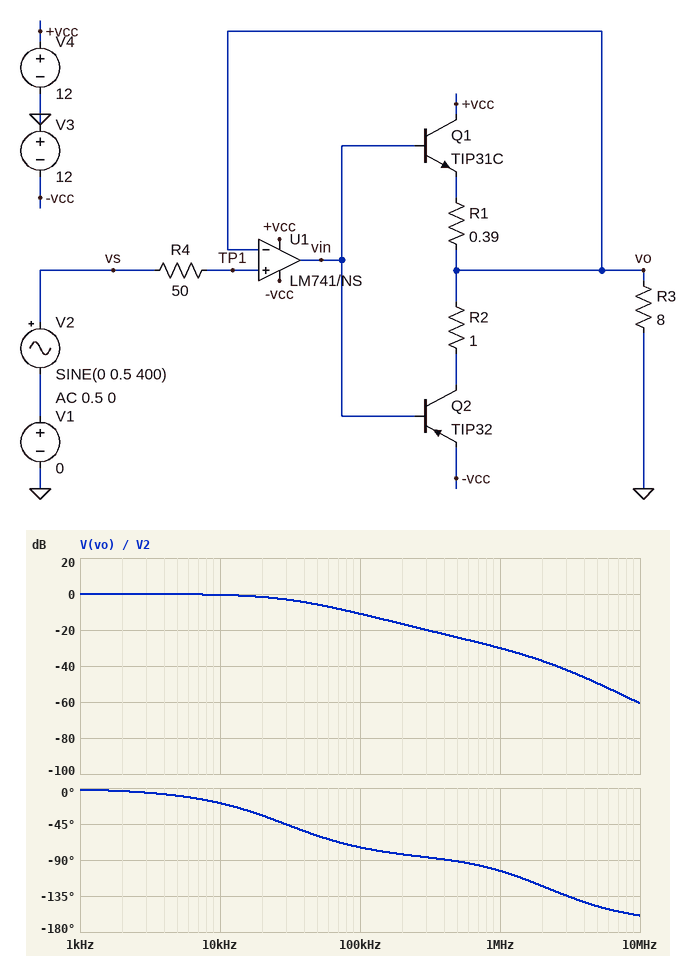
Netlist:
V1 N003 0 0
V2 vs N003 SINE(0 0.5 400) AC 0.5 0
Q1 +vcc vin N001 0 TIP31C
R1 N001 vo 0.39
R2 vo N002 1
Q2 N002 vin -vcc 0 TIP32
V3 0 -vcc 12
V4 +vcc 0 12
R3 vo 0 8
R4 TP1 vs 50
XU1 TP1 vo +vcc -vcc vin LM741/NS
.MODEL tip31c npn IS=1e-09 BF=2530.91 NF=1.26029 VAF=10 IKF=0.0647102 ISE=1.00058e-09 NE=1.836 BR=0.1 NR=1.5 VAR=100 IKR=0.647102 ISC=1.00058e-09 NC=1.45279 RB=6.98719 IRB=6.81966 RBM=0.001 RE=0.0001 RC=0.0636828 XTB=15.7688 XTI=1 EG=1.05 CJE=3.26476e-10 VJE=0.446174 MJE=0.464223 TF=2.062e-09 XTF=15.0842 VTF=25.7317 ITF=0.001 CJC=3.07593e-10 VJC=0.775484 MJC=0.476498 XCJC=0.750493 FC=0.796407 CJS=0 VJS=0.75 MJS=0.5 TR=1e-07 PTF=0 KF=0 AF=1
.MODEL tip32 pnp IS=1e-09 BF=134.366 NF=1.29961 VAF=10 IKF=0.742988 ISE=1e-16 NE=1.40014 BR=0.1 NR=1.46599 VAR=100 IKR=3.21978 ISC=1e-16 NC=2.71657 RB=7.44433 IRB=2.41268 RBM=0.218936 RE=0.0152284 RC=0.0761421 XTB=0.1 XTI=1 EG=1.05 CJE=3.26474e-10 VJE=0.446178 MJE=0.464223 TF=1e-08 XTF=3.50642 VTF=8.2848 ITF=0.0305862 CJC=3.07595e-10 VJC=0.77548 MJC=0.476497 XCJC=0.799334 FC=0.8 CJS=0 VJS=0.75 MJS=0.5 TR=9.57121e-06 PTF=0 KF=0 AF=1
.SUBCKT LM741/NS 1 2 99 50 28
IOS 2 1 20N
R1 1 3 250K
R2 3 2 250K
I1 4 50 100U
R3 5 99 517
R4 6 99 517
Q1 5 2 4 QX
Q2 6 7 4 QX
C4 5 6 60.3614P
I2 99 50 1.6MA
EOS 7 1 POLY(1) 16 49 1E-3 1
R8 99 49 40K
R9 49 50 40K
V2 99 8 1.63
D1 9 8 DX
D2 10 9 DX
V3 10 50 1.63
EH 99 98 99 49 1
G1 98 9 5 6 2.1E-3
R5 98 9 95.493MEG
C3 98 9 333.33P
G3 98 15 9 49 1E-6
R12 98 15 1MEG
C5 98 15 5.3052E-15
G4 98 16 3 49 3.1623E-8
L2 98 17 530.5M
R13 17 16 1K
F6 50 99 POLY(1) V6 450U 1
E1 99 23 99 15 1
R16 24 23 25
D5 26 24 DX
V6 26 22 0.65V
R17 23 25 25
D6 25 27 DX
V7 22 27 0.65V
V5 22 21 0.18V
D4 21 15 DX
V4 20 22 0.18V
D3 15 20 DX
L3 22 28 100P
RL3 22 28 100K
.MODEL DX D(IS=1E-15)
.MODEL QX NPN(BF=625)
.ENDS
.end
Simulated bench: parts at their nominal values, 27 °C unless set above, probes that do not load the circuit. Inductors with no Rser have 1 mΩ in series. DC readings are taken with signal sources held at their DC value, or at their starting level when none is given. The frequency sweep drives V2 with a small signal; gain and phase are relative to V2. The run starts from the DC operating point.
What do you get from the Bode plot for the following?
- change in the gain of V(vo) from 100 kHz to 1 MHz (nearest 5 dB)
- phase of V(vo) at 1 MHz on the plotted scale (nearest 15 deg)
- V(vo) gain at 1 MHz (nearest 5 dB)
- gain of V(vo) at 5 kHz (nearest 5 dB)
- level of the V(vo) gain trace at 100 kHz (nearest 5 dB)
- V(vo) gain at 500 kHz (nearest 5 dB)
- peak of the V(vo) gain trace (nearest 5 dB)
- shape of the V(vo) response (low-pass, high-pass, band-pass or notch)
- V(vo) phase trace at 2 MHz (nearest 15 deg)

-20 dB
-105 deg
-30 dB
0 dB
-10 dB
-25 dB
0 dB
low-pass
-120 deg
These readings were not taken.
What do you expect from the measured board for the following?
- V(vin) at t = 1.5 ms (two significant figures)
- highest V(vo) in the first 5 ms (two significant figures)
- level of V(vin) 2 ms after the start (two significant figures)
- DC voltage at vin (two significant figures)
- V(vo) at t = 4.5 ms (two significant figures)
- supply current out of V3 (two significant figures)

-990 mV
500 mV
-990 mV
360 mV
-220 mV
1.6 mA
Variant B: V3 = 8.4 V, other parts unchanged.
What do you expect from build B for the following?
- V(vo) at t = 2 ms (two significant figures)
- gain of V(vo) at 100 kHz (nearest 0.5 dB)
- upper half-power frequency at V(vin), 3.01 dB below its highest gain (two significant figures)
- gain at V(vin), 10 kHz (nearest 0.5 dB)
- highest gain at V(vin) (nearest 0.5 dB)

-220 mV
-11.5 dB
28 kHz
30.5 dB
31.0 dB
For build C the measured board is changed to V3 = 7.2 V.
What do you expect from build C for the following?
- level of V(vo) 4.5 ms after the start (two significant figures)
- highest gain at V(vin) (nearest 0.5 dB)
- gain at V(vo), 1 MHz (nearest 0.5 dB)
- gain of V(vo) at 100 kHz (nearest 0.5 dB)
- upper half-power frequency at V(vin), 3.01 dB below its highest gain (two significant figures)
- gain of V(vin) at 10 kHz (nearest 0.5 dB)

-210 mV
31.0 dB
-30.5 dB
-11.5 dB
27 kHz
30.5 dB
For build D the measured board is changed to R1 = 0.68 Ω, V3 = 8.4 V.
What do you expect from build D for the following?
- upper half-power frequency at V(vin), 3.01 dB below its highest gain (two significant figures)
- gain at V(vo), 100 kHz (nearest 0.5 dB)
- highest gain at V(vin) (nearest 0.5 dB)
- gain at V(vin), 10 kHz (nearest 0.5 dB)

28 kHz
-11.5 dB
31.0 dB
30.5 dB
